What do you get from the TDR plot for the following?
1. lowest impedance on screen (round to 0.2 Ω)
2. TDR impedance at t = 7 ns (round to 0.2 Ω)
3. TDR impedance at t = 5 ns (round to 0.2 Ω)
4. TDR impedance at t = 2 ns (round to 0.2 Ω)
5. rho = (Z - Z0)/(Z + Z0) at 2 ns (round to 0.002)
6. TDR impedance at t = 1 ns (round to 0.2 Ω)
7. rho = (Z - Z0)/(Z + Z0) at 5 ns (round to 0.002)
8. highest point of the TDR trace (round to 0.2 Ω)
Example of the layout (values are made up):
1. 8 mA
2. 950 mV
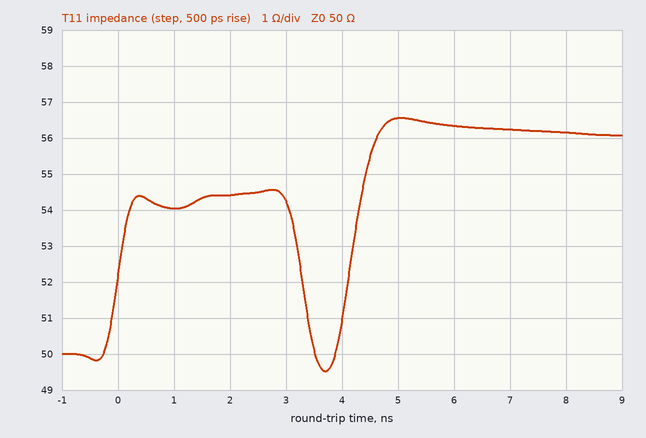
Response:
1. 49.6 Ω
2. 56.2 Ω
3. 56.6 Ω
4. 54.4 Ω
5. +0.042
6. 54.0 Ω
7. +0.062
8. 56.6 Ω
